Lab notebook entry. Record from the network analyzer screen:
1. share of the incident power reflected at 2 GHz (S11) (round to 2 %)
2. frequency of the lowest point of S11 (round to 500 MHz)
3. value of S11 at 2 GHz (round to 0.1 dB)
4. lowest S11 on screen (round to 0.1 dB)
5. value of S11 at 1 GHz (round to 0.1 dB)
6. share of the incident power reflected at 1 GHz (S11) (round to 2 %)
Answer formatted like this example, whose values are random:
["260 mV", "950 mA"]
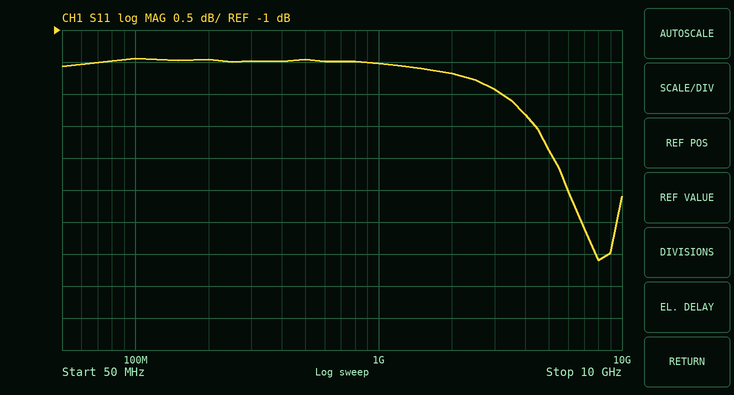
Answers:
["68 %", "8.0 GHz", "-1.7 dB", "-4.6 dB", "-1.5 dB", "70 %"]
